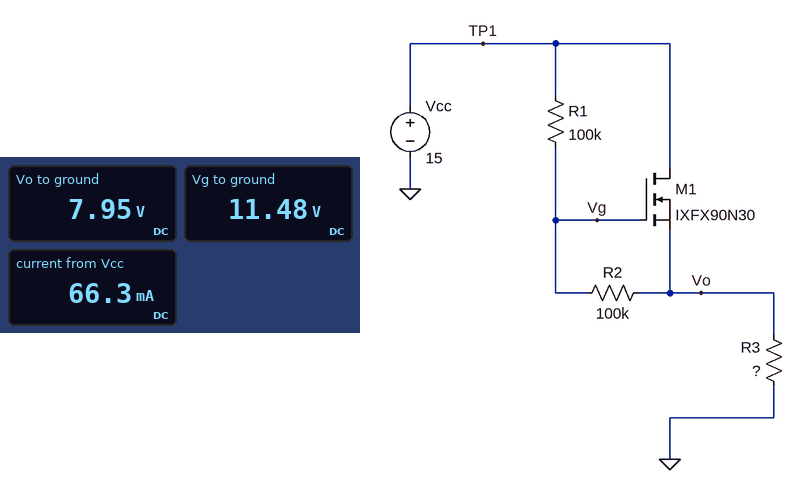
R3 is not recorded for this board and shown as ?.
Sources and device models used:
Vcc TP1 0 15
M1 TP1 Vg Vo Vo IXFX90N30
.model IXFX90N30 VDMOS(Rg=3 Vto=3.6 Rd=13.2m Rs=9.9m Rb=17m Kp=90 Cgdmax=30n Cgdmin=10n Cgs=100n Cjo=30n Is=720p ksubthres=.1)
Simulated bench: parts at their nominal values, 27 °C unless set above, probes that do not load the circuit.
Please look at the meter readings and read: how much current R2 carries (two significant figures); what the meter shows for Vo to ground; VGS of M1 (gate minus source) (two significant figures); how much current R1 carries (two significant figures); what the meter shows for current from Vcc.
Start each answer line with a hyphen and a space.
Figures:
- 35 µA
- 7.95 V
- 3.5 V
- 35 µA
- 66.3 mA
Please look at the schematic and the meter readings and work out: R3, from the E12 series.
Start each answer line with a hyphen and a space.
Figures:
- 120 Ω
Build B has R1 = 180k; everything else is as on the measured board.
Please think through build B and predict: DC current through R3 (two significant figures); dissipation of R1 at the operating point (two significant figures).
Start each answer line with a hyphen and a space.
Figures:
- 43 mA
- 220 µW
